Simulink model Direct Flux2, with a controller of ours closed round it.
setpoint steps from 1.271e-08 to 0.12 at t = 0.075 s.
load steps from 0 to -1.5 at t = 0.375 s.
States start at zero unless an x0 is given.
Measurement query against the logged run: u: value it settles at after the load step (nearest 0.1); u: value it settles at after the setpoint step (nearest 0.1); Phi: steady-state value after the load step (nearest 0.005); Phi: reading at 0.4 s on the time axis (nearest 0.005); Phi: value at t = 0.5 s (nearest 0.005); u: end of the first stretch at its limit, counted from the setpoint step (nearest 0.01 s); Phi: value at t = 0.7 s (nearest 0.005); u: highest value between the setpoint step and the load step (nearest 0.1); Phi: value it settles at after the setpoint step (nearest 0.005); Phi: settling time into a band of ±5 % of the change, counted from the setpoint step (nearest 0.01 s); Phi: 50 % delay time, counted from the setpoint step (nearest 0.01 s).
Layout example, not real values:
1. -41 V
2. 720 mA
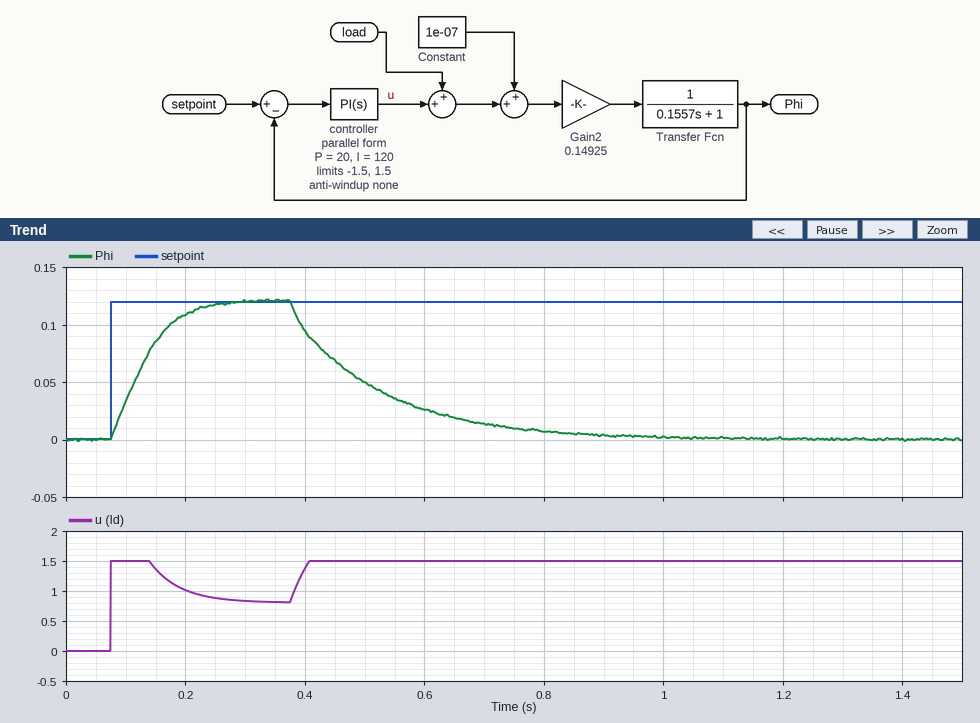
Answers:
1. 1.5
2. 0.8
3. 0.000
4. 0.095
5. 0.050
6. 0.07 s
7. 0.015
8. 1.5
9. 0.120
10. 0.15 s
11. 0.05 s
